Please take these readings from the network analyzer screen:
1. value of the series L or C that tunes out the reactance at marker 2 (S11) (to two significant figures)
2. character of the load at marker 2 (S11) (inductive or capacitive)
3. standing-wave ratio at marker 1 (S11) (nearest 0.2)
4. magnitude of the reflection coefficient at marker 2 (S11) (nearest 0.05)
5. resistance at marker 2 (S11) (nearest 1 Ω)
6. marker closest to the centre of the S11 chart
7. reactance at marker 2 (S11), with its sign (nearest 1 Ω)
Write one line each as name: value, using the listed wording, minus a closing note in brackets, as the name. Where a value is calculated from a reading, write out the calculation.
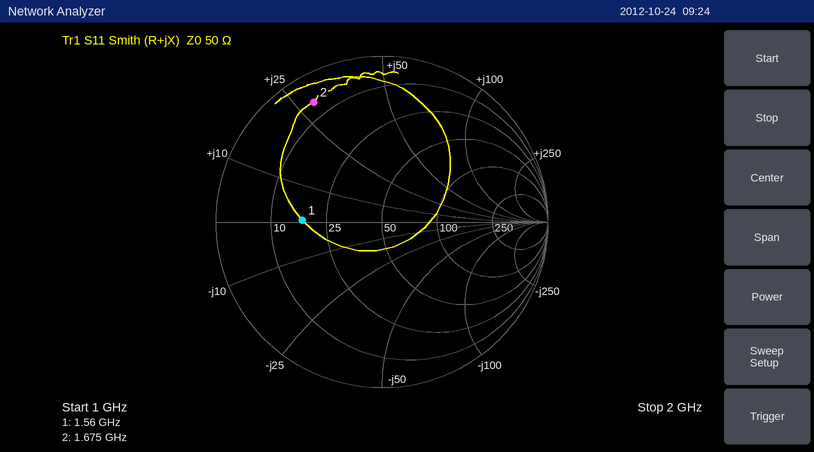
value of the series L or C that tunes out the reactance at marker 2 (S11): C = 1/(2π × 1.675 GHz × 29 Ω) ≈ 3.3 pF
character of the load at marker 2 (S11): inductive
standing-wave ratio at marker 1 (S11): 2.8
magnitude of the reflection coefficient at marker 2 (S11): 0.85
resistance at marker 2 (S11): 6 Ω
marker closest to the centre of the S11 chart: marker 1
reactance at marker 2 (S11), with its sign: +29 Ω
